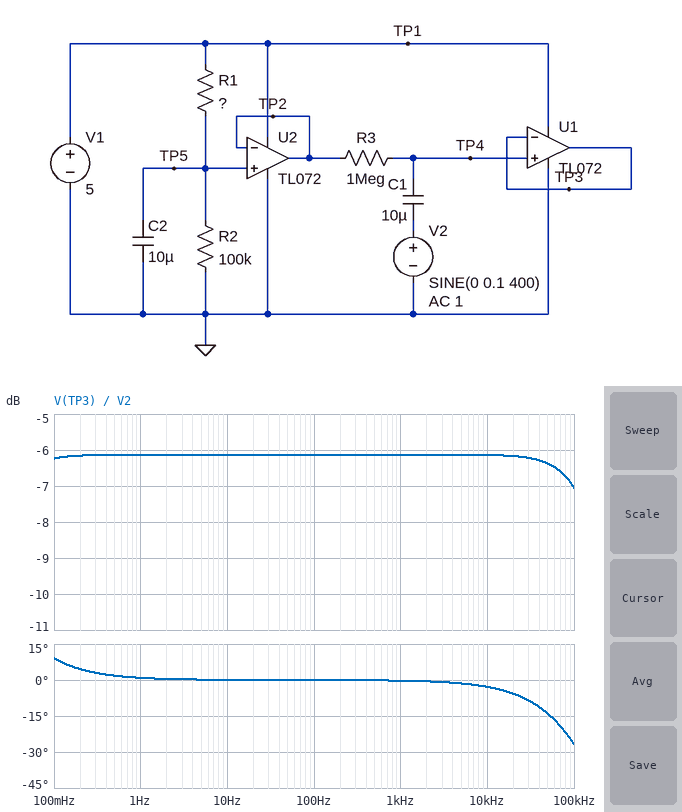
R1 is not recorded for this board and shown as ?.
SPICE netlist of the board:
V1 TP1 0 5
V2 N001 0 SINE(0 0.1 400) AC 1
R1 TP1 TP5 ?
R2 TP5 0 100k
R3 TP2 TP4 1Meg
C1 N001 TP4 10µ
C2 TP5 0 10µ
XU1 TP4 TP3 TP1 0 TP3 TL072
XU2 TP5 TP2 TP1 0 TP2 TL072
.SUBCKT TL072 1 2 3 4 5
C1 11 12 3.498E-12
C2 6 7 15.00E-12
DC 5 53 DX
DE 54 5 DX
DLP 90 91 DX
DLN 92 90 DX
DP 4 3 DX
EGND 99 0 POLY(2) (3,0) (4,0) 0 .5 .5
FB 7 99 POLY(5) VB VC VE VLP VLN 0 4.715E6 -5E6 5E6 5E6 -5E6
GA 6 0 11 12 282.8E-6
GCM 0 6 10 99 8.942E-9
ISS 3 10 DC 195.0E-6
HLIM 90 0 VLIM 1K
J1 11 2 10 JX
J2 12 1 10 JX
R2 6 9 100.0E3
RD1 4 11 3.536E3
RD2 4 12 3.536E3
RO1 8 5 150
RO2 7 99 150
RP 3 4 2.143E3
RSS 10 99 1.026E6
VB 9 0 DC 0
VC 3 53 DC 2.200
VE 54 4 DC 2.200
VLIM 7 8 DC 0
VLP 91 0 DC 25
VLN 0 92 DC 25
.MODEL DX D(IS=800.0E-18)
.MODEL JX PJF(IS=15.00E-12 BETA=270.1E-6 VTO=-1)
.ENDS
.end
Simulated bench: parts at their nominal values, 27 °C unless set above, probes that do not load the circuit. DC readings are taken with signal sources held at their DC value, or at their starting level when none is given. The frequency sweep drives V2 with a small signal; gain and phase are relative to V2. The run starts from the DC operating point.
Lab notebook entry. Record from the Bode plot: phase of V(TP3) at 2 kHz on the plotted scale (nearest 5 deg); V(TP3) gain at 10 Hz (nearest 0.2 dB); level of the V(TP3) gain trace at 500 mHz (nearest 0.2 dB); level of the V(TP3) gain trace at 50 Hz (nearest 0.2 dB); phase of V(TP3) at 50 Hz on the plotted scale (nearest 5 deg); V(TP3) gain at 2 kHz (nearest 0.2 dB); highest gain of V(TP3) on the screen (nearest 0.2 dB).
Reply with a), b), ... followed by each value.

a) 0 deg
b) -6.2 dB
c) -6.2 dB
d) -6.2 dB
e) 0 deg
f) -6.2 dB
g) -6.2 dB
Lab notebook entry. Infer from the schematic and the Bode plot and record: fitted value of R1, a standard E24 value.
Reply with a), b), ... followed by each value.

a) 43 kΩ
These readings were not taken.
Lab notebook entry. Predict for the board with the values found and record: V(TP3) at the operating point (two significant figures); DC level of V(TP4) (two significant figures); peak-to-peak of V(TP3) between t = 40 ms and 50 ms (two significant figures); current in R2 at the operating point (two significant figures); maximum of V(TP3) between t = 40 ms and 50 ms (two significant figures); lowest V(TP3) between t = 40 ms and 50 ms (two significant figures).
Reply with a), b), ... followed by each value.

a) 3.4 V
b) 3.4 V
c) 110 mV
d) 35 µA
e) 3.4 V
f) 3.3 V
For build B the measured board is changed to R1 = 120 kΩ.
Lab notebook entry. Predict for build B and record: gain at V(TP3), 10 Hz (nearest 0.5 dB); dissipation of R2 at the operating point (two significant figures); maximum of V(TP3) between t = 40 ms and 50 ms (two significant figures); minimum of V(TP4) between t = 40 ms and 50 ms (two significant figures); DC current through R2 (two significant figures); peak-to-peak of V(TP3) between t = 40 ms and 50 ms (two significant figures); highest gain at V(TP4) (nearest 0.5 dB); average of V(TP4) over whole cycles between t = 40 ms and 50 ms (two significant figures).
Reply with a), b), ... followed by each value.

a) 0 dB
b) 52 µW
c) 2.4 V
d) 2.2 V
e) 23 µA
f) 200 mV
g) 0 dB
h) 2.3 V
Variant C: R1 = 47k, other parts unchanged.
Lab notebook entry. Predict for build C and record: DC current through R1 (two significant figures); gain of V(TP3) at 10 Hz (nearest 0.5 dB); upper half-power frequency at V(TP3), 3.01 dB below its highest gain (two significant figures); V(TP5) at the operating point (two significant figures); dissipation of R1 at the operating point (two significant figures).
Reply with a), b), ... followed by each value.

a) 34 µA
b) -3.0 dB
c) 340 kHz
d) 3.4 V
e) 54 µW
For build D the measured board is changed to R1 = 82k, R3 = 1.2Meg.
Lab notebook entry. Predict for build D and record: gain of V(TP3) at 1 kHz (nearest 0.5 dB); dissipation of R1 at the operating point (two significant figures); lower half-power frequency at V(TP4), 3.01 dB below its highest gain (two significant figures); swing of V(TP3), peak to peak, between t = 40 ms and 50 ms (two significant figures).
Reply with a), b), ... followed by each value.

a) 0 dB
b) 62 µW
c) 13 mHz
d) 200 mV
